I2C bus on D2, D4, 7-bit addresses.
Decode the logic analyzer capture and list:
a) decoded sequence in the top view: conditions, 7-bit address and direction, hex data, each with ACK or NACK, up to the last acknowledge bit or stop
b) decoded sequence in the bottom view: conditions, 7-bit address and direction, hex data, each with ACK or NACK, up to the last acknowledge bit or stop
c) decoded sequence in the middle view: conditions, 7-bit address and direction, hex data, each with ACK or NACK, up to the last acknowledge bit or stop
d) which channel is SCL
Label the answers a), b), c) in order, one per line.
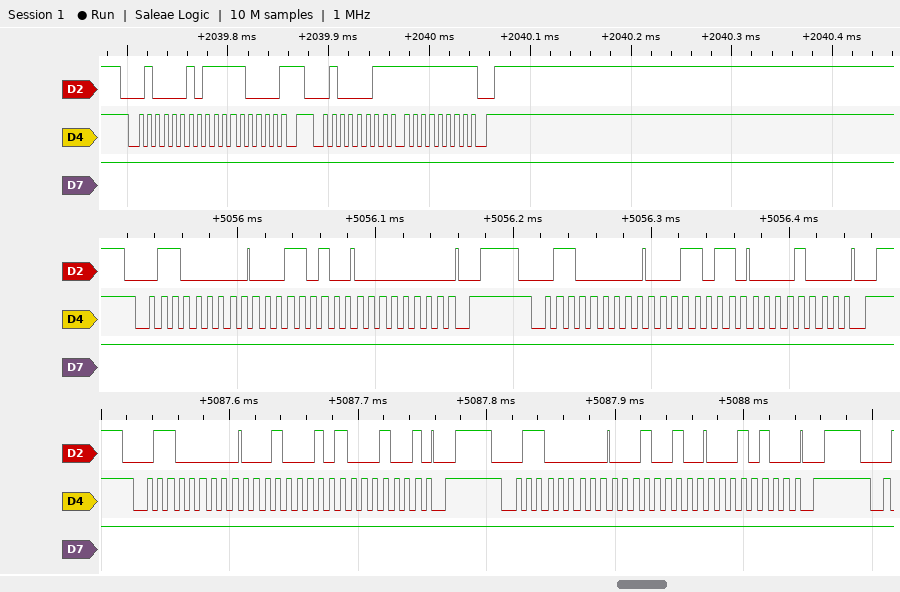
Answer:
a) start, address 21 write NACK, F0 NACK, repeated start, address 21 read NACK, FF NACK, stop
b) start, address 30 write ACK, 11 ACK, 89 ACK, stop, start, address 30 write ACK, 12 ACK, 14 ACK, stop
c) start, address 30 write ACK, 1A ACK, 00 ACK, stop, start, address 30 write ACK, 1B ACK, 08 ACK, stop
d) D4
